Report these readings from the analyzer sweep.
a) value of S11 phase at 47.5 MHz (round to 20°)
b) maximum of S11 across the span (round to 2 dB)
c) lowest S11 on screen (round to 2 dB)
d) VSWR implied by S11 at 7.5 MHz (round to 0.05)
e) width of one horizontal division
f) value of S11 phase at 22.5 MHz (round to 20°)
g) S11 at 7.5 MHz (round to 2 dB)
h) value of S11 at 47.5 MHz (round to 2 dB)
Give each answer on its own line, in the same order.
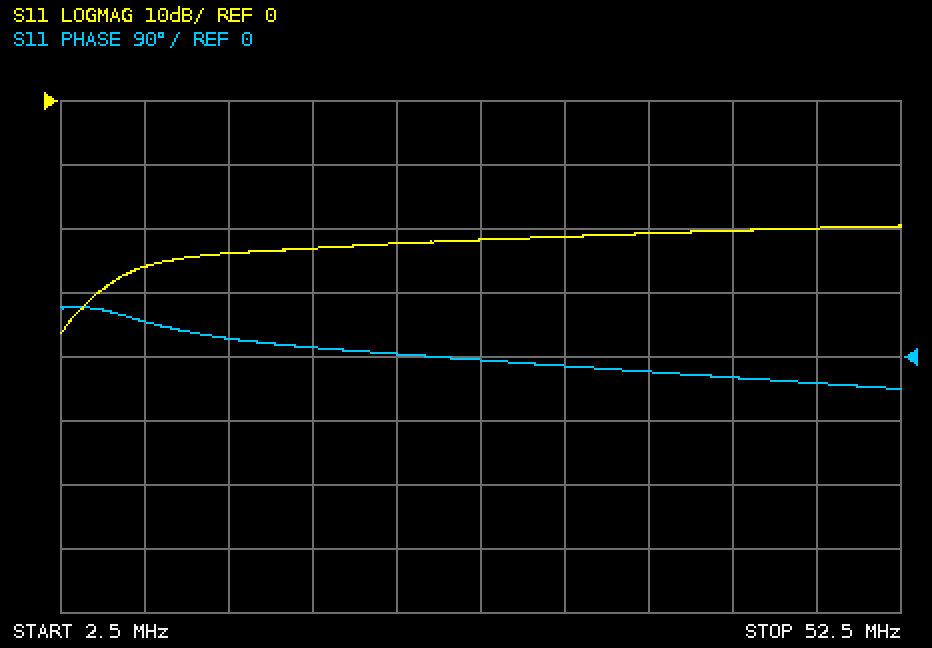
-40°
-20 dB
-36 dB
1.10
5 MHz
0°
-26 dB
-20 dB
